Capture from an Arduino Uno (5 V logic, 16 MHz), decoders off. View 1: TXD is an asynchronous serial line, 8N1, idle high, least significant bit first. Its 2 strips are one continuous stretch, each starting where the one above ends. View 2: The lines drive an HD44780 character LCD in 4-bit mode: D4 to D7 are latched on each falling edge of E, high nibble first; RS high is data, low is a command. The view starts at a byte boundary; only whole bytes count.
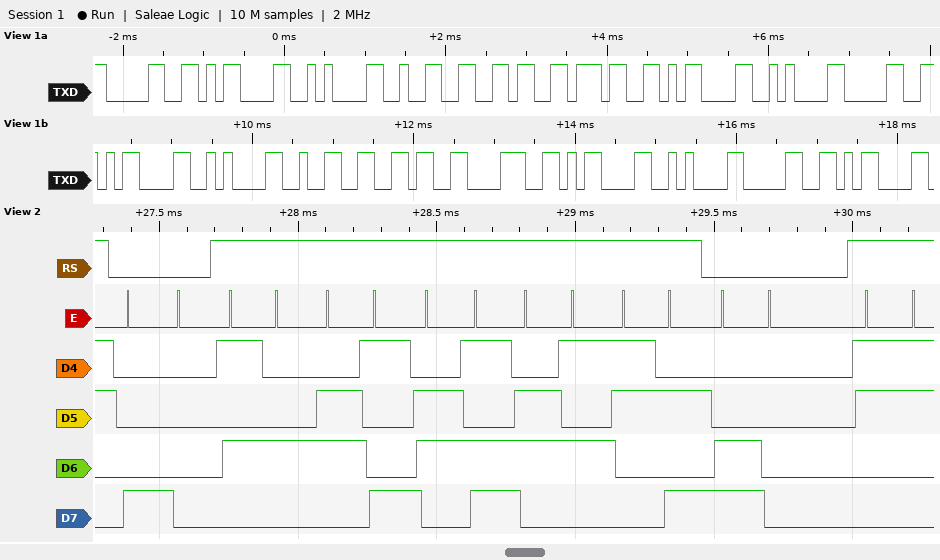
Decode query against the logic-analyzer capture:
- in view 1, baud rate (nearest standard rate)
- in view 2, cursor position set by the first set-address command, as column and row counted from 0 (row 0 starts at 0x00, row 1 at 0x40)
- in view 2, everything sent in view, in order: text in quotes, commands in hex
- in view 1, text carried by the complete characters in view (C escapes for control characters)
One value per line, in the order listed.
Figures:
9600 baud
column 0, row 0
0x80 "Time:" 0xC0 "3"
"0\r\n267\r\n0\r\n268\r\n0\r"
